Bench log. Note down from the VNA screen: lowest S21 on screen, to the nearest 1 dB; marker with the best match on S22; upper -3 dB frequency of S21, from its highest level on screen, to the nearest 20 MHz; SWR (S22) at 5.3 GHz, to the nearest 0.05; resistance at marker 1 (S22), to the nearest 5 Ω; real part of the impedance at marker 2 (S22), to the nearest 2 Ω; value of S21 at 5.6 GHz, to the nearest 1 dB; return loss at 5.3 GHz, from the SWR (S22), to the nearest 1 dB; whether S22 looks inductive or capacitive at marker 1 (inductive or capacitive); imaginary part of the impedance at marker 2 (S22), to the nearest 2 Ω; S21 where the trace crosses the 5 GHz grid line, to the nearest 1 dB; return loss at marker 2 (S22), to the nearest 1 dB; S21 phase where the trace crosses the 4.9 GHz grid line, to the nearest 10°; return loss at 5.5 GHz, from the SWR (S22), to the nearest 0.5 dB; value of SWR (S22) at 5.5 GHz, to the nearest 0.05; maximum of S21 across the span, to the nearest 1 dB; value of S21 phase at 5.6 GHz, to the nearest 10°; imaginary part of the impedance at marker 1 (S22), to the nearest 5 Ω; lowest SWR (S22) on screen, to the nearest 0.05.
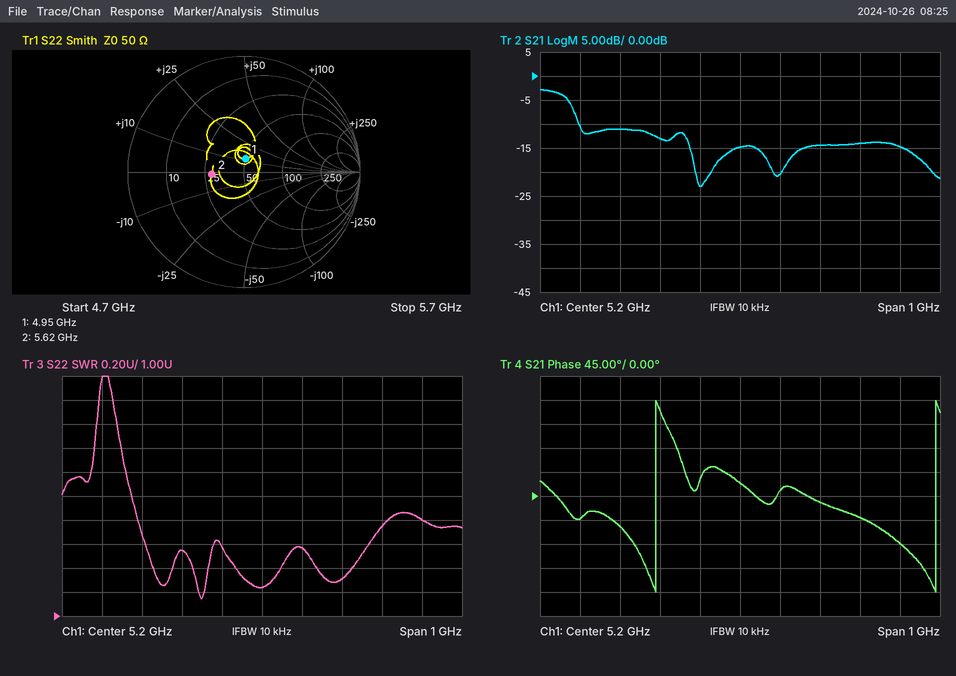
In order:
-23 dB
marker 1
4.78 GHz
1.55
50 Ω
28 Ω
-15 dB
13 dB
inductive
-2 Ω
-13 dB
11 dB
-60°
11.5 dB
1.75
-3 dB
-90°
+10 Ω
1.15
